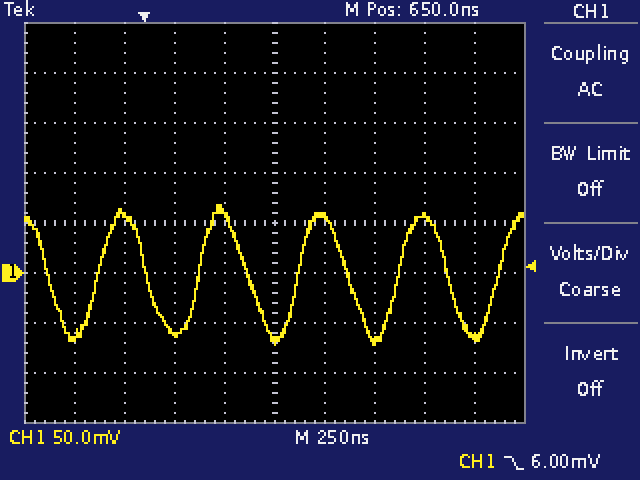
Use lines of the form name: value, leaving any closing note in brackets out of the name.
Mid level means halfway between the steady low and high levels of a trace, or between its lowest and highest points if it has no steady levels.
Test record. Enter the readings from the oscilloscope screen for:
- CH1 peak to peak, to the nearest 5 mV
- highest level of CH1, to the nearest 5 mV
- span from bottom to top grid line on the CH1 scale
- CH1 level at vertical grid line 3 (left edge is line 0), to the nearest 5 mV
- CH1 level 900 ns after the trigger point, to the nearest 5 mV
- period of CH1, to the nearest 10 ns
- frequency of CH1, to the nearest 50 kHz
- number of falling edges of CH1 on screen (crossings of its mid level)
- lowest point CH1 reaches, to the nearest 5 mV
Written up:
CH1 peak to peak, to the nearest 5 mV: 140 mV
highest level of CH1, to the nearest 5 mV: 70 mV
span from bottom to top grid line on the CH1 scale: 400 mV
CH1 level at vertical grid line 3 (left edge is line 0), to the nearest 5 mV: -60 mV
CH1 level 900 ns after the trigger point, to the nearest 5 mV: 55 mV
period of CH1, to the nearest 10 ns: 500 ns
frequency of CH1, to the nearest 50 kHz: 2.00 MHz
number of falling edges of CH1 on screen: 5
lowest point CH1 reaches, to the nearest 5 mV: -70 mV
